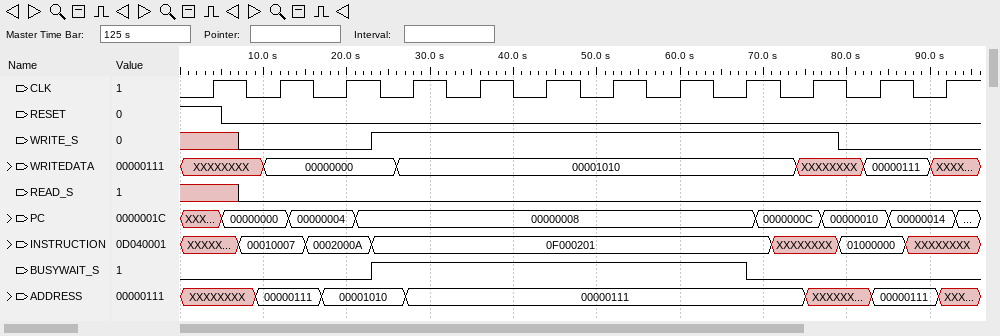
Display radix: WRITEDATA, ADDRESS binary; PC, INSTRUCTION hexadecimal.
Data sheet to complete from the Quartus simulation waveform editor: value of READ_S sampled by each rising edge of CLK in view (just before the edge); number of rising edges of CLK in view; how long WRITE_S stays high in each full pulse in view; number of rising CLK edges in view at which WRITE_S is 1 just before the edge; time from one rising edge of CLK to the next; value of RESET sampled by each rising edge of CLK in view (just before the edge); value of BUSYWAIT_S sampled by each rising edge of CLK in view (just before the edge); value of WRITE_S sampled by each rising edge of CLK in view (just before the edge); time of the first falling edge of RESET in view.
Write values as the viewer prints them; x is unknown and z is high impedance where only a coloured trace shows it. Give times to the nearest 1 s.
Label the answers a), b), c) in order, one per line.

a) x 0 0 0 0 0 0 0 0 0 0 0
b) 12
c) 56 s
d) 7
e) 8 s
f) 1 0 0 0 0 0 0 0 0 0 0 0
g) 0 0 0 1 1 1 1 1 1 0 0 0
h) x 0 0 1 1 1 1 1 1 1 0 0
i) 5 s
